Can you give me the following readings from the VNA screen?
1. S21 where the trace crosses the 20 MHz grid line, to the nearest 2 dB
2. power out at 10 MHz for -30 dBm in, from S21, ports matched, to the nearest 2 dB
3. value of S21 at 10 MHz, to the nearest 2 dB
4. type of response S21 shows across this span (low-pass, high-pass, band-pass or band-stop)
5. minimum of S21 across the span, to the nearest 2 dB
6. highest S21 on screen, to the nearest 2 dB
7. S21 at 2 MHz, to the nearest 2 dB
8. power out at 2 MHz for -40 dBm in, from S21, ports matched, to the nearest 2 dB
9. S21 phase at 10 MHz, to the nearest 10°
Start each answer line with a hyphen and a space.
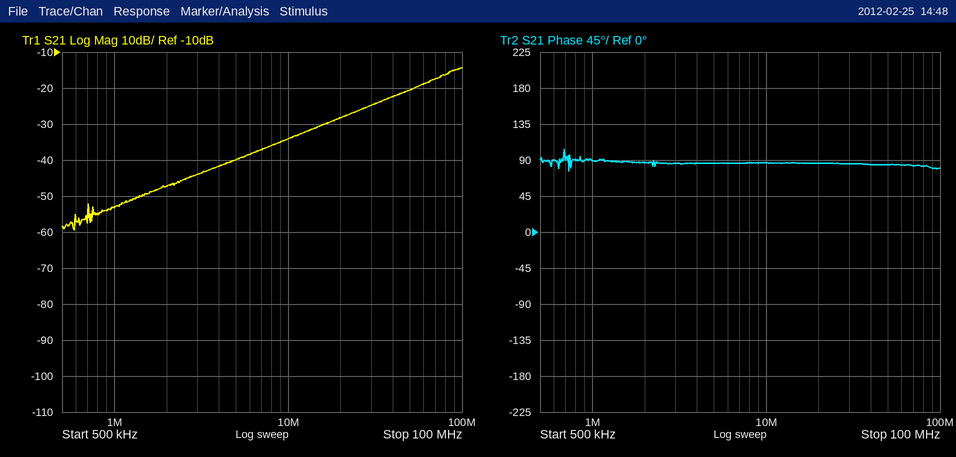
- -28 dB
- -64 dBm
- -34 dB
- high-pass
- -60 dB
- -14 dB
- -48 dB
- -88 dBm
- 90°
